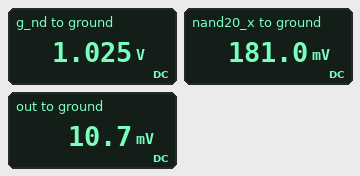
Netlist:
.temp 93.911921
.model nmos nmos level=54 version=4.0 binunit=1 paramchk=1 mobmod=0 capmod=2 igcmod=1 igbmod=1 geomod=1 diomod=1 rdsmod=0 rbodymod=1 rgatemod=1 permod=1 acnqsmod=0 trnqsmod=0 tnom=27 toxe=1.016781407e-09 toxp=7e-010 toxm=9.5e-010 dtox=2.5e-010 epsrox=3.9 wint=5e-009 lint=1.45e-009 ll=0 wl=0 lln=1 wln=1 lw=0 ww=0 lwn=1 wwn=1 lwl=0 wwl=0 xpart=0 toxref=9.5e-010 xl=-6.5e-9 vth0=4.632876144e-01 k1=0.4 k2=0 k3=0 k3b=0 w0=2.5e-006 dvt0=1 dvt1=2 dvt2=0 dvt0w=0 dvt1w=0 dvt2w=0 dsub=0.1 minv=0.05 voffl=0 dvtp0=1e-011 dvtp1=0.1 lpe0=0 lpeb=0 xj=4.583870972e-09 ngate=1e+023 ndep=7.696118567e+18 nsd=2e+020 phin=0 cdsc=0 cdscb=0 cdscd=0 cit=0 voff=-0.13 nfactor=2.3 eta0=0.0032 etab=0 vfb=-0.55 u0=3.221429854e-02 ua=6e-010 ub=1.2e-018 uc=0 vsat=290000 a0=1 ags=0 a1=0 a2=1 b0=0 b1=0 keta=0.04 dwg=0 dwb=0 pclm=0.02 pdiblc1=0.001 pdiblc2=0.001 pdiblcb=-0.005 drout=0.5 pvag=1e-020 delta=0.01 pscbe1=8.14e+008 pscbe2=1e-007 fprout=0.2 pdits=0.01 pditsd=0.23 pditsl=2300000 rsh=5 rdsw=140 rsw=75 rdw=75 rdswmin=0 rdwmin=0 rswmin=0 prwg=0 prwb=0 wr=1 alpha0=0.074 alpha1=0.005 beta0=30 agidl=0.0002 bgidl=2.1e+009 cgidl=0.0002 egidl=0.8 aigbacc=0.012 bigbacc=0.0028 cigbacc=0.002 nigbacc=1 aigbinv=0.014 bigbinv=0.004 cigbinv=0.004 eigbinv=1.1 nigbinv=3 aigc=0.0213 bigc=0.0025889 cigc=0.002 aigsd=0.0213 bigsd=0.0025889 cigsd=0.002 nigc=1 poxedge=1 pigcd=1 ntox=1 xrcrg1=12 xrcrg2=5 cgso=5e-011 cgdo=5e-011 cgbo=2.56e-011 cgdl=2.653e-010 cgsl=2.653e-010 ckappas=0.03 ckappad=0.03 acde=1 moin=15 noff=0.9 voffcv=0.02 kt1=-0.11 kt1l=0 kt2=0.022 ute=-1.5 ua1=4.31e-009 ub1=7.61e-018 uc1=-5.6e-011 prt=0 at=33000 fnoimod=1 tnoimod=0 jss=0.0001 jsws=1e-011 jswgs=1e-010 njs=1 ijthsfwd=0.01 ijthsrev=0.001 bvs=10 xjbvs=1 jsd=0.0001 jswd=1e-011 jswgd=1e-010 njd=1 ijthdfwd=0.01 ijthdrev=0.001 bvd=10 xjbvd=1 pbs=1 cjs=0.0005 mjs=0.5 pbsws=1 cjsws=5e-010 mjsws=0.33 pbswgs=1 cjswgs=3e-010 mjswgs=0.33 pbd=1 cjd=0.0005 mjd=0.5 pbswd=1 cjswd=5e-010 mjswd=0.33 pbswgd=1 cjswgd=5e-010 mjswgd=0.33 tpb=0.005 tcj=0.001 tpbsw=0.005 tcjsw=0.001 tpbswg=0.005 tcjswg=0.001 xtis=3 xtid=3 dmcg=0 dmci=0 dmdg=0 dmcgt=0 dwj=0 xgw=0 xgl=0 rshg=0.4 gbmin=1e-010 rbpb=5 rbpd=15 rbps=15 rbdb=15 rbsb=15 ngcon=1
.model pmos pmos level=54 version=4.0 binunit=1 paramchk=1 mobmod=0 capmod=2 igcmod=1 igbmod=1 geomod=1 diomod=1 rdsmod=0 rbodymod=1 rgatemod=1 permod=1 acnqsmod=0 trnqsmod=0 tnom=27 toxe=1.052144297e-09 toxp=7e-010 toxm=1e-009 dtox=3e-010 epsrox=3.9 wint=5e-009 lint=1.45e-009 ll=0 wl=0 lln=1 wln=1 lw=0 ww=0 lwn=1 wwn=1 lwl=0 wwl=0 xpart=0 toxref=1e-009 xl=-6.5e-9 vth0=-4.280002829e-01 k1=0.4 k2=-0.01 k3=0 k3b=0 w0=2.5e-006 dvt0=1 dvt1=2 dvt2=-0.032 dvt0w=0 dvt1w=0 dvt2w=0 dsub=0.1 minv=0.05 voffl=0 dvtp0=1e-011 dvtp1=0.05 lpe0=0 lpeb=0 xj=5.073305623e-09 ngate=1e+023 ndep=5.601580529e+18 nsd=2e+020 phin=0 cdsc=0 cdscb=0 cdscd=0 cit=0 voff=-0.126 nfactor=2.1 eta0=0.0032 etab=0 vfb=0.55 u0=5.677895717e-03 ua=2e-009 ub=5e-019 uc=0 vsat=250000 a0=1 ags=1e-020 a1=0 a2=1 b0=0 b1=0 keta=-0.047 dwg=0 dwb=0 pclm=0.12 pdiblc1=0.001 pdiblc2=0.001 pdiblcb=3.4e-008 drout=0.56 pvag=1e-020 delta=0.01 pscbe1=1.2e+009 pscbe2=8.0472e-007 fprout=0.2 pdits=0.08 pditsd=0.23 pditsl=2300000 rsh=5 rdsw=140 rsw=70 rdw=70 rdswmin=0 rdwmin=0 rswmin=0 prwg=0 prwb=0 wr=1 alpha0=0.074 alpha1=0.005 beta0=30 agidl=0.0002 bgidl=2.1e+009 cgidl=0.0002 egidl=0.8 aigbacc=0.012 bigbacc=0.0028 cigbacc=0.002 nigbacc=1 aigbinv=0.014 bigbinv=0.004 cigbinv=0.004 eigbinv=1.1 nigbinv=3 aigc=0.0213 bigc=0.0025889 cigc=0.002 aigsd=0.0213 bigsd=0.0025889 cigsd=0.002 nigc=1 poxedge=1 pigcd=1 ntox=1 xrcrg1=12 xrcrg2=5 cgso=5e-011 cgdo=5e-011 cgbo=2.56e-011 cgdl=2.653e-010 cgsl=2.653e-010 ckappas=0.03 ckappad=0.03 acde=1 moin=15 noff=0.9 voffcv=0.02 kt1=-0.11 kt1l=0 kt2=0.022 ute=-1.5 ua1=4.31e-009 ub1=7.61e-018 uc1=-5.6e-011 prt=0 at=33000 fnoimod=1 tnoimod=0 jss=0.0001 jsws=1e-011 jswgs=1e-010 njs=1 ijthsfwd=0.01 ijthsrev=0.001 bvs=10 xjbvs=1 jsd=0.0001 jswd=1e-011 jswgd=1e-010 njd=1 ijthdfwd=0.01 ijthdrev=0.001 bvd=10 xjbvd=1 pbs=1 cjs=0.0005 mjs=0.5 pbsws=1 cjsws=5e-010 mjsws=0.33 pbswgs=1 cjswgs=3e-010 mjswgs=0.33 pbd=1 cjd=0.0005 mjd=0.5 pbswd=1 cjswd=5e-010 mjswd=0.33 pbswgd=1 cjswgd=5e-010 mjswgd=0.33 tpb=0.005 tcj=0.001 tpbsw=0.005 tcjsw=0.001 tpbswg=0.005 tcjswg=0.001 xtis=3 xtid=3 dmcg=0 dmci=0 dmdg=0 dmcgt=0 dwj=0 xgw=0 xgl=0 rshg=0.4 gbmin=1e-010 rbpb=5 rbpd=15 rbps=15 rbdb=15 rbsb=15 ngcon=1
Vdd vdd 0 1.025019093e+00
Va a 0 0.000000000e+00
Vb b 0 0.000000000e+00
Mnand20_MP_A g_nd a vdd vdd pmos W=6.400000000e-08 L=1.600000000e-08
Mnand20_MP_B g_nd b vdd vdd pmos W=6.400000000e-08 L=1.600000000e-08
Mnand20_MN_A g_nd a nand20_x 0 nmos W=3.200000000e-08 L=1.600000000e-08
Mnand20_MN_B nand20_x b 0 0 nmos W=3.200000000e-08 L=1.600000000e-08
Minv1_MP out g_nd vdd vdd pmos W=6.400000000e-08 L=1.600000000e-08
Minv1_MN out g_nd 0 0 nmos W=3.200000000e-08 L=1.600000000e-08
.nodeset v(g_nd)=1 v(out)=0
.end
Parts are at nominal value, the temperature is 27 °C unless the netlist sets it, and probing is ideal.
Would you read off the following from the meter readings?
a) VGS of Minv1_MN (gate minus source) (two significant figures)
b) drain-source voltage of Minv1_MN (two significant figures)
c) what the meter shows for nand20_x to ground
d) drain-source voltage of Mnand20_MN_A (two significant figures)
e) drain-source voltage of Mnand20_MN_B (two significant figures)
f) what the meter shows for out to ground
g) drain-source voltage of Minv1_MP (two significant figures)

1.0 V
11 mV
181.0 mV
840 mV
180 mV
10.7 mV
-1.0 V
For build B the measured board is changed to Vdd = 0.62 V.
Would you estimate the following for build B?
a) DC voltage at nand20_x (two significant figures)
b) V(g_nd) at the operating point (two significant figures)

110 mV
620 mV
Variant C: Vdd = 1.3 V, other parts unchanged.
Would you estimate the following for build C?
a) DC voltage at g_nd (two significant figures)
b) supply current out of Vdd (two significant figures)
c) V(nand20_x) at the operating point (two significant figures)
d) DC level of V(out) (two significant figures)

1.3 V
8.8 µA
240 mV
78 mV
